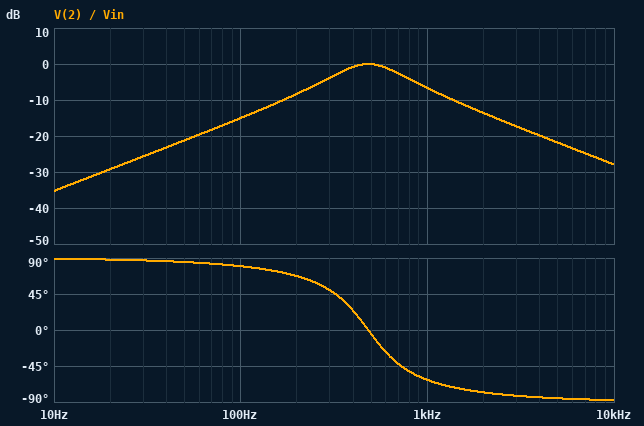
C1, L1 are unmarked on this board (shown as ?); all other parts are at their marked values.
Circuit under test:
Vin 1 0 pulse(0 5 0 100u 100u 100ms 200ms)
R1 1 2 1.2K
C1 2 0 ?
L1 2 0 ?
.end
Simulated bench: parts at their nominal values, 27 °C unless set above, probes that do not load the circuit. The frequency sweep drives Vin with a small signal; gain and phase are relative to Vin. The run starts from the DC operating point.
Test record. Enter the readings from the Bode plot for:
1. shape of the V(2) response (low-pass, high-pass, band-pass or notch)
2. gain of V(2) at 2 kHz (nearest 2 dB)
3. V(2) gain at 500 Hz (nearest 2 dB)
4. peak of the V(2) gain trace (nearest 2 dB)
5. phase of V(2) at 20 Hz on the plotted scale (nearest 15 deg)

band-pass
-14 dB
0 dB
0 dB
90 deg
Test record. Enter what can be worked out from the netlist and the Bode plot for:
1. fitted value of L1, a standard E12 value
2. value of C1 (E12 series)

330 mH
330 nF
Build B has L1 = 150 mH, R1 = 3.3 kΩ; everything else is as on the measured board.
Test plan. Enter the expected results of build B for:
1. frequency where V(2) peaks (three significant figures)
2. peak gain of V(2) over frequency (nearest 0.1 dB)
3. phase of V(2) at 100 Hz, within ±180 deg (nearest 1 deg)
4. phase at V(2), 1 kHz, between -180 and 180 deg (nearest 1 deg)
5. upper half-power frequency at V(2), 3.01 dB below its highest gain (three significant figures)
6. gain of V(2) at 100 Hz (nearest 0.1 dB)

715 Hz
0 dB
88 deg
-73 deg
792 Hz
-30.7 dB
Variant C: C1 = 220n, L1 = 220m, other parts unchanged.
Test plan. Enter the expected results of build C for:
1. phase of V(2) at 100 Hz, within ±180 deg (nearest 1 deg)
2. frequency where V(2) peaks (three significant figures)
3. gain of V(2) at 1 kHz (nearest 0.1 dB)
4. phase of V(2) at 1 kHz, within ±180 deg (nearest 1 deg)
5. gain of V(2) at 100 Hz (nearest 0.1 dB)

83 deg
723 Hz
-2.1 dB
-38 deg
-18.7 dB
